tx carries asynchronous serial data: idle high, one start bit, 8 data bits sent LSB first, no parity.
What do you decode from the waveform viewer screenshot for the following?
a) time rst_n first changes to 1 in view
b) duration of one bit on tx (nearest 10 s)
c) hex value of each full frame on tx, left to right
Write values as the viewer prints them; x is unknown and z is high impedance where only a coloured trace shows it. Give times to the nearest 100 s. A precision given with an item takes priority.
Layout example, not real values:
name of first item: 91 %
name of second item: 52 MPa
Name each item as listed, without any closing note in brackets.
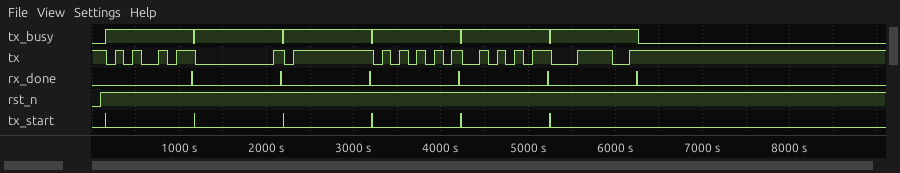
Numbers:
time rst_n first changes to 1 in view: 100 s
duration of one bit on tx: 100 s
hex value of each full frame on tx, left to right: A5, 00, FF, 55, AA, 3C
